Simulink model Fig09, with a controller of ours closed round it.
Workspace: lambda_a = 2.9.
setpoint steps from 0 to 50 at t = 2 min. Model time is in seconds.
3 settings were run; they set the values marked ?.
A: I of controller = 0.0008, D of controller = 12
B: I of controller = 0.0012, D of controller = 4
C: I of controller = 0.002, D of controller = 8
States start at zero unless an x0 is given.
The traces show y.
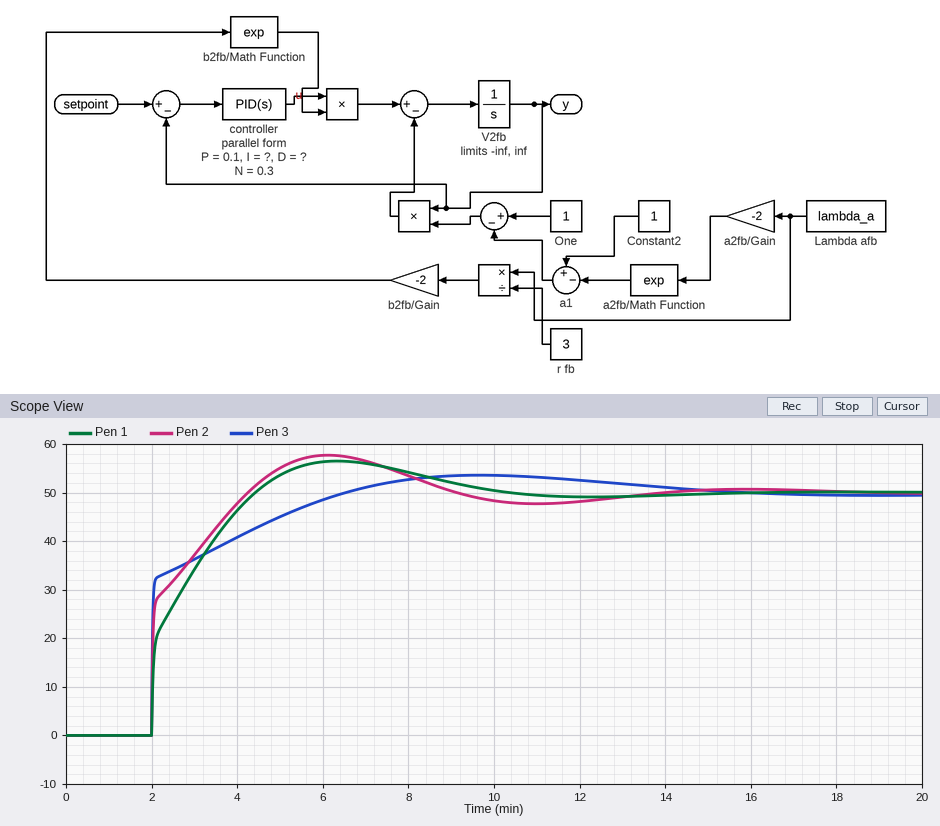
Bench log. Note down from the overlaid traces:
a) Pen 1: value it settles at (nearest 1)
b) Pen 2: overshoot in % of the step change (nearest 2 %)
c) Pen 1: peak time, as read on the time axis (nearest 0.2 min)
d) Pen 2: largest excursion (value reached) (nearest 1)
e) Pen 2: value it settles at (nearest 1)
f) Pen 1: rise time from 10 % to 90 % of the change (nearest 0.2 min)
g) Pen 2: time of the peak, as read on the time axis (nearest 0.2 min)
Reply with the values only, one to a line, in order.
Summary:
50
16 %
6.4 min
58
50
1.8 min
6.2 min
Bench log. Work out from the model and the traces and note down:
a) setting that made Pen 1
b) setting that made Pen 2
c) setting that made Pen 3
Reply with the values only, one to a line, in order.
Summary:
B
C
A
